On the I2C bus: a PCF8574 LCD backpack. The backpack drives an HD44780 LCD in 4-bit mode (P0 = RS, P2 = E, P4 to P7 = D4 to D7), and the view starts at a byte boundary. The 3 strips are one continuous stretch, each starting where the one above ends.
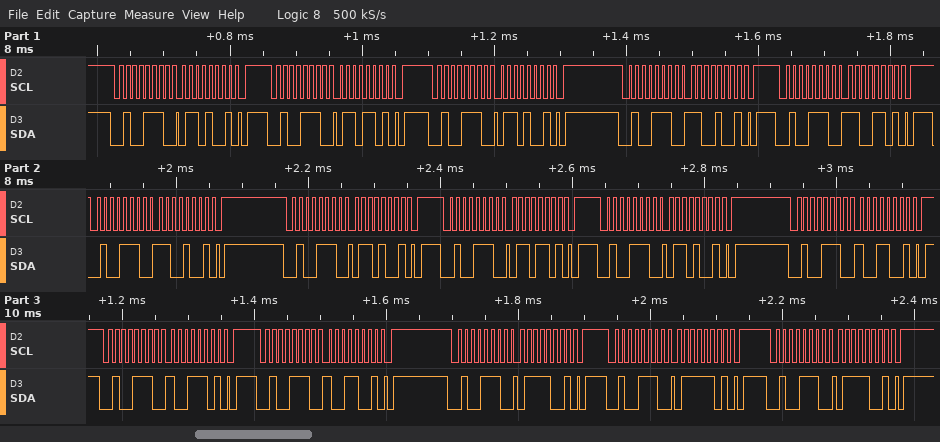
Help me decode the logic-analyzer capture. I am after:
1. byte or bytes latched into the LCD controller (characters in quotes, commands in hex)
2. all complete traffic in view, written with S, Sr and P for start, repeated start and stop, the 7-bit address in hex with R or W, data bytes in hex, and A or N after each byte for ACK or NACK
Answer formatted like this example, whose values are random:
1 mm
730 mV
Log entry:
'l' 'i'
S 27W A 69 A P S 27W A 6D A P S 27W A 69 A P S 27W A C9 A P S 27W A CD A P S 27W A C9 A P S 27W A 69 A P S 27W A 6D A P S 27W A 69 A P S 27W A 99 A P S 27W A 9D A P S 27W A 99 A P S 27W A 79 A P S 27W A 7D A P S 27W A 79 A P
